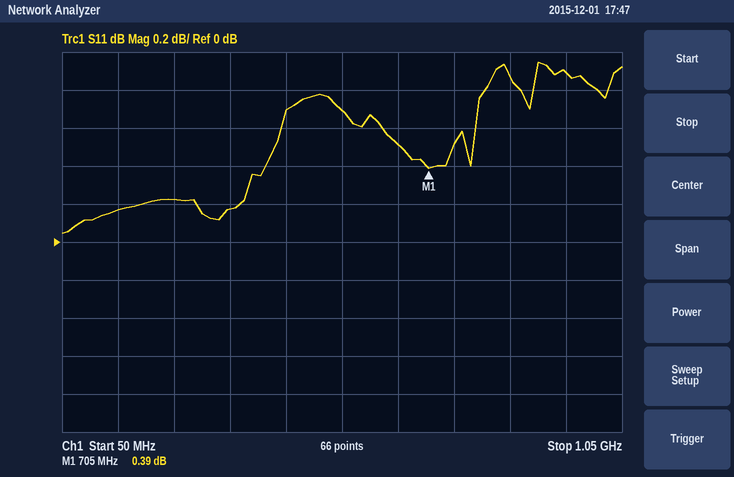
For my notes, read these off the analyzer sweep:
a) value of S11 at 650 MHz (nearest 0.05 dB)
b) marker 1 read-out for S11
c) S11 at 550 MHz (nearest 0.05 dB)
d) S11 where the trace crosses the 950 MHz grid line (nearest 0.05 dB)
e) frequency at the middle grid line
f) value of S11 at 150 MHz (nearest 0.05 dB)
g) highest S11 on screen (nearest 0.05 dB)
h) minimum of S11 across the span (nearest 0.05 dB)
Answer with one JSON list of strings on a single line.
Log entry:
["0.50 dB", "0.39 dB", "0.70 dB", "0.90 dB", "550 MHz", "0.15 dB", "0.95 dB", "0.05 dB"]
